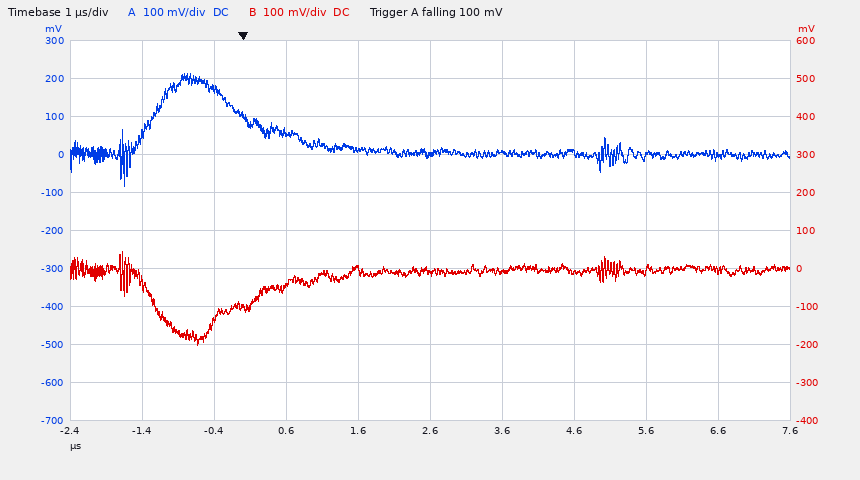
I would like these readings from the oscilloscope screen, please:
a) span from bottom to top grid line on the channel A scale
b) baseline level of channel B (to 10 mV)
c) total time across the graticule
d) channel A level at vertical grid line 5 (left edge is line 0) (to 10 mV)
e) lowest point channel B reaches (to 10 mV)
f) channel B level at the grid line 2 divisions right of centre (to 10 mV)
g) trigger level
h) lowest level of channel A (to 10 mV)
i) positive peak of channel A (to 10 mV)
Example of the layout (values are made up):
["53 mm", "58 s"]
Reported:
["1 V", "-10 mV", "10 µs", "0 mV", "-200 mV", "-10 mV", "100 mV", "-80 mV", "210 mV"]
